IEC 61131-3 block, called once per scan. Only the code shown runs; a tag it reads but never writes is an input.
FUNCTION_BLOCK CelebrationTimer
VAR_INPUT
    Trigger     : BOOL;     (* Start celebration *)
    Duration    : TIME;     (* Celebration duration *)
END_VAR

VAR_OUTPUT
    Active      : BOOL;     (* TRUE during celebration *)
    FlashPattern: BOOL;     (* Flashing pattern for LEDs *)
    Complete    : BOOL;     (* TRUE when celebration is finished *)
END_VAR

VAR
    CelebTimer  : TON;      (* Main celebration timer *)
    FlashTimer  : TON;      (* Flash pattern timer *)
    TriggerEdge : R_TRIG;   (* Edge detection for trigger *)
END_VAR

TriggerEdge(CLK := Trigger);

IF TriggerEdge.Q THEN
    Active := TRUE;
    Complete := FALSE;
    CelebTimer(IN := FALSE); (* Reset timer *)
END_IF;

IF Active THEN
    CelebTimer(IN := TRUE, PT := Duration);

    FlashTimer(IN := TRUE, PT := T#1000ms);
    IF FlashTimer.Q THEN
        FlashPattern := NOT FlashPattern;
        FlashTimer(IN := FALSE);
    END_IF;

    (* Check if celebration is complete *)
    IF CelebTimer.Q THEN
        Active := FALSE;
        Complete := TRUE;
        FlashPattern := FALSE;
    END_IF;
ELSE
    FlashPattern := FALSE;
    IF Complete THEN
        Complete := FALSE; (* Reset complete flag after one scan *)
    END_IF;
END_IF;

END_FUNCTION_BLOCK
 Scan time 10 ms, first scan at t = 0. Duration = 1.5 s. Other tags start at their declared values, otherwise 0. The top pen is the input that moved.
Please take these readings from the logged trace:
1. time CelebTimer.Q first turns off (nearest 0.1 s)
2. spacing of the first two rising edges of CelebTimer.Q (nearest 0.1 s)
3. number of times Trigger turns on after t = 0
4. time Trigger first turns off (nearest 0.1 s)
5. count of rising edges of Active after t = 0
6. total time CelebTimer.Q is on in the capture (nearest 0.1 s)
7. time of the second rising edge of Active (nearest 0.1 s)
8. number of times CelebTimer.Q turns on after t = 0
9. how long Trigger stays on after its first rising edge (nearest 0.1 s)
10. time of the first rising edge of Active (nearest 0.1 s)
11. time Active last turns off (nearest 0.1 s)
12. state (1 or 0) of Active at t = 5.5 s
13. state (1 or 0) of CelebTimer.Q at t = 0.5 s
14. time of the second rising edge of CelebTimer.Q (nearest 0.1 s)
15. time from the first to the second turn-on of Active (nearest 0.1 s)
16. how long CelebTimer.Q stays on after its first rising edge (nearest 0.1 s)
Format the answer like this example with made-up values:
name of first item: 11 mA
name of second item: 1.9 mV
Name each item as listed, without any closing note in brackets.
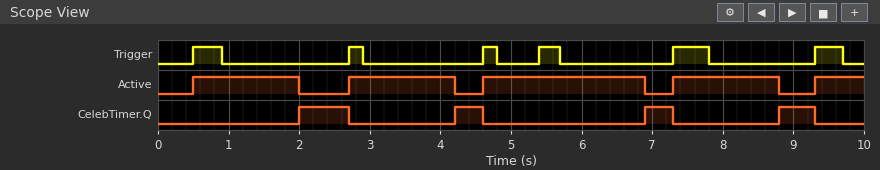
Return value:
time CelebTimer.Q first turns off: 2.7 s
spacing of the first two rising edges of CelebTimer.Q: 2.2 s
number of times Trigger turns on after t = 0: 6
time Trigger first turns off: 0.9 s
count of rising edges of Active after t = 0: 5
total time CelebTimer.Q is on in the capture: 2.0 s
time of the second rising edge of Active: 2.7 s
number of times CelebTimer.Q turns on after t = 0: 4
how long Trigger stays on after its first rising edge: 0.4 s
time of the first rising edge of Active: 0.5 s
time Active last turns off: 8.8 s
state (1 or 0) of Active at t = 5.5 s: 1
state (1 or 0) of CelebTimer.Q at t = 0.5 s: 0
time of the second rising edge of CelebTimer.Q: 4.2 s
time from the first to the second turn-on of Active: 2.2 s
how long CelebTimer.Q stays on after its first rising edge: 0.7 s
